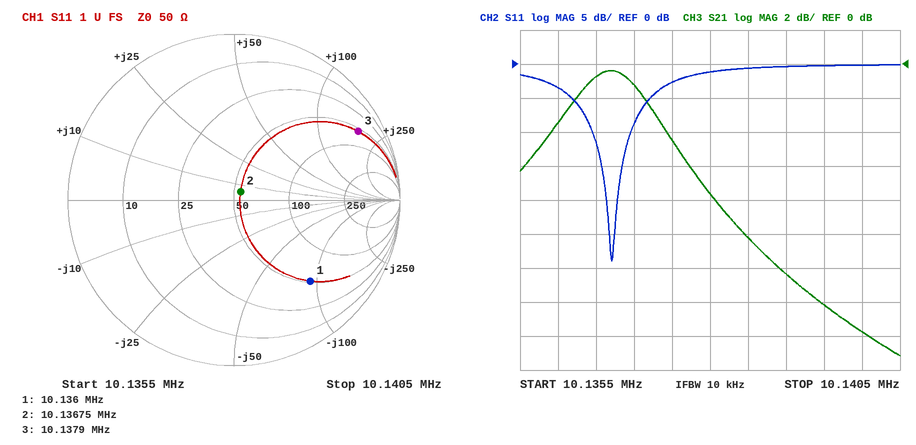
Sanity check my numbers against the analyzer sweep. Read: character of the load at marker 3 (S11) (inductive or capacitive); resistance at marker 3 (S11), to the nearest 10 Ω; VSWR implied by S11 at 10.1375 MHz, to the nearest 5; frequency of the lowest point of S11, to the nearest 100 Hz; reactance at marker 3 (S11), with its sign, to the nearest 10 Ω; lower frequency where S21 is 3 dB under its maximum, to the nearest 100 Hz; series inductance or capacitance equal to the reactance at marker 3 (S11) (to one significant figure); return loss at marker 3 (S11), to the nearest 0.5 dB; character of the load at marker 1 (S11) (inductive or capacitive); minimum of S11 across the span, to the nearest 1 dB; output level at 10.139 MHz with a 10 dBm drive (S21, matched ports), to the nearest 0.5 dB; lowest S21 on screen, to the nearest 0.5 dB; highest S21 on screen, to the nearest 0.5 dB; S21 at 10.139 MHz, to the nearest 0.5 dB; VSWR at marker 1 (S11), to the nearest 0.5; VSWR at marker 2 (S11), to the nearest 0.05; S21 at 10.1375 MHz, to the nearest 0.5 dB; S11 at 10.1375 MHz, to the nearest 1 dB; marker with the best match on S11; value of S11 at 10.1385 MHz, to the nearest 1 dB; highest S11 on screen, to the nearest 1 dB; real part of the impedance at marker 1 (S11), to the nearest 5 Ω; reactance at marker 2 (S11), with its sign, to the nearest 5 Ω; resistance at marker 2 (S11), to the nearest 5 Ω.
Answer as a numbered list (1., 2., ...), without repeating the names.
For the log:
1. inductive
2. 60 Ω
3. 5
4. 10.1367 MHz
5. +180 Ω
6. 10.1360 MHz
7. 3 µH
8. 1.5 dB
9. capacitive
10. -29 dB
11. -2.5 dBm
12. -17.0 dB
13. -0.5 dB
14. -12.5 dB
15. 5.0
16. 1.15
17. -4.5 dB
18. -3 dB
19. marker 2
20. -1 dB
21. 0 dB
22. 50 Ω
23. +5 Ω
24. 55 Ω
